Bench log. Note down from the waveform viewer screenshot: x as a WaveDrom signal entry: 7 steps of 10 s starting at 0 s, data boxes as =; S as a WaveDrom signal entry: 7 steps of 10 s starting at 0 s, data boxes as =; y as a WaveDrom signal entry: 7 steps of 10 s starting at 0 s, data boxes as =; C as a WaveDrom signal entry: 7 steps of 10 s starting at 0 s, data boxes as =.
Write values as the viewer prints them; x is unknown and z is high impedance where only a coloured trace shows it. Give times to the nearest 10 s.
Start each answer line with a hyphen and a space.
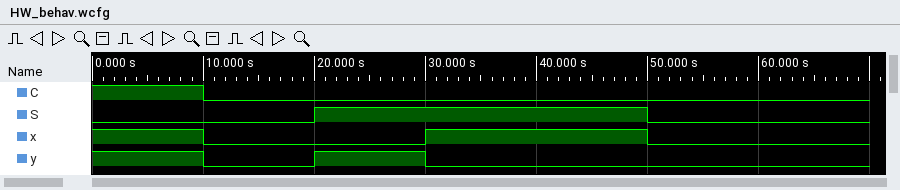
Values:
- {name: 'x', wave: '10.1.0.'}
- {name: 'S', wave: '0.1..0.'}
- {name: 'y', wave: '1010...'}
- {name: 'C', wave: '10.....'}
